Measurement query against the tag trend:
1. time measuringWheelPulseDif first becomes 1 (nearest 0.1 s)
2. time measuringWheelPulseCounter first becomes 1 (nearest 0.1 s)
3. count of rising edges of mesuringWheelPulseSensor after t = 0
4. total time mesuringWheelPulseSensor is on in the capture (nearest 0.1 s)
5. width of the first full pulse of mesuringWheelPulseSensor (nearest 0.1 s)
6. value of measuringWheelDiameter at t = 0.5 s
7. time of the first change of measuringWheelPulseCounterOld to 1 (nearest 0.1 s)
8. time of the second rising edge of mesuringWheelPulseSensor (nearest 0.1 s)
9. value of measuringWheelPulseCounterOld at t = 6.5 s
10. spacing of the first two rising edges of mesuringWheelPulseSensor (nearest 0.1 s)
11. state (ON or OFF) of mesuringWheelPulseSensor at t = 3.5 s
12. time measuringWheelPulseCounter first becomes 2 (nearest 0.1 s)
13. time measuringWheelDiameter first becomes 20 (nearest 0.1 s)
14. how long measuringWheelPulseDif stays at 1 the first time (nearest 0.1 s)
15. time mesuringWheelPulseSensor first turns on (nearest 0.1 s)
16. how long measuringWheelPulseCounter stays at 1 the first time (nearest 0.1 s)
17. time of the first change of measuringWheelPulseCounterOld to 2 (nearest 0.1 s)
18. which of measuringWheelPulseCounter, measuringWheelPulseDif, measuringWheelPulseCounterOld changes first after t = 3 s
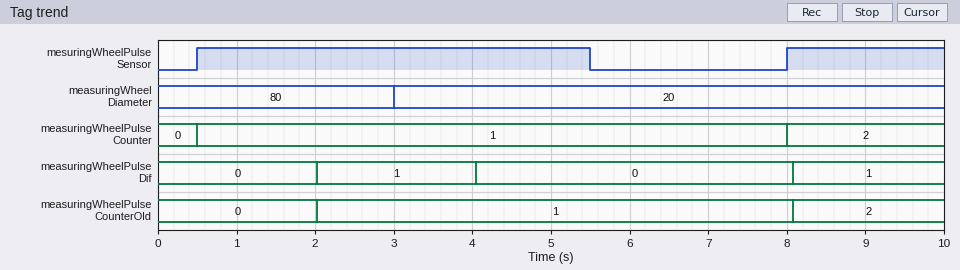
2.0 s
0.5 s
2
7.0 s
5.0 s
80
2.0 s
8.0 s
1
7.5 s
ON
8.0 s
3.0 s
2.0 s
0.5 s
7.5 s
8.1 s
measuringWheelPulseDif
